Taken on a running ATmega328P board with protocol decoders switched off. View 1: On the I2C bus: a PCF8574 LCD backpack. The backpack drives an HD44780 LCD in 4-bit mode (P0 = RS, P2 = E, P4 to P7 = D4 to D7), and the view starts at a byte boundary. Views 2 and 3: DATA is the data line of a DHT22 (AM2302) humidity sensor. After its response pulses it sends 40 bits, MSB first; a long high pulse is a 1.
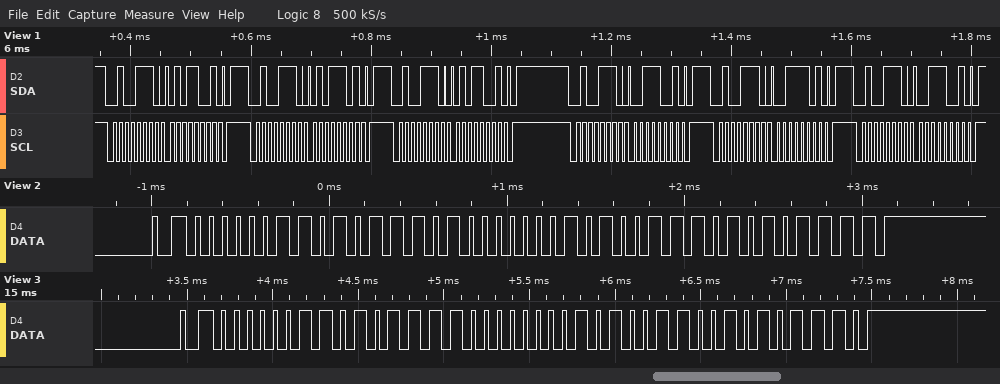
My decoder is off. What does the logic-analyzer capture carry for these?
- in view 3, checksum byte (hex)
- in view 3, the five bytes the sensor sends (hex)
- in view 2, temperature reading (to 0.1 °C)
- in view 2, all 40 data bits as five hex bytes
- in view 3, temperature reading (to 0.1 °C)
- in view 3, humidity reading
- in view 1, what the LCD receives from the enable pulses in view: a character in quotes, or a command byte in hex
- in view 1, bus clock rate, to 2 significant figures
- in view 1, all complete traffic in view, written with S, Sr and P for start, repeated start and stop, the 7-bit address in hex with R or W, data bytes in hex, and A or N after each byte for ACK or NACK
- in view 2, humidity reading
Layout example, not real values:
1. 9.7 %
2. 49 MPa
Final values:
1. 0xAE
2. 03 5E 01 4C AE
3. 33.4 °C
4. 03 5D 01 4E AF
5. 33.2 °C
6. 86.2 %
7. 'S'
8. 100 kHz
9. S 27W A 59 A P S 27W A 5D A P S 27W A 59 A P S 27W A 39 A P S 27W A 3D A P S 27W A 39 A P
10. 86.1 %
